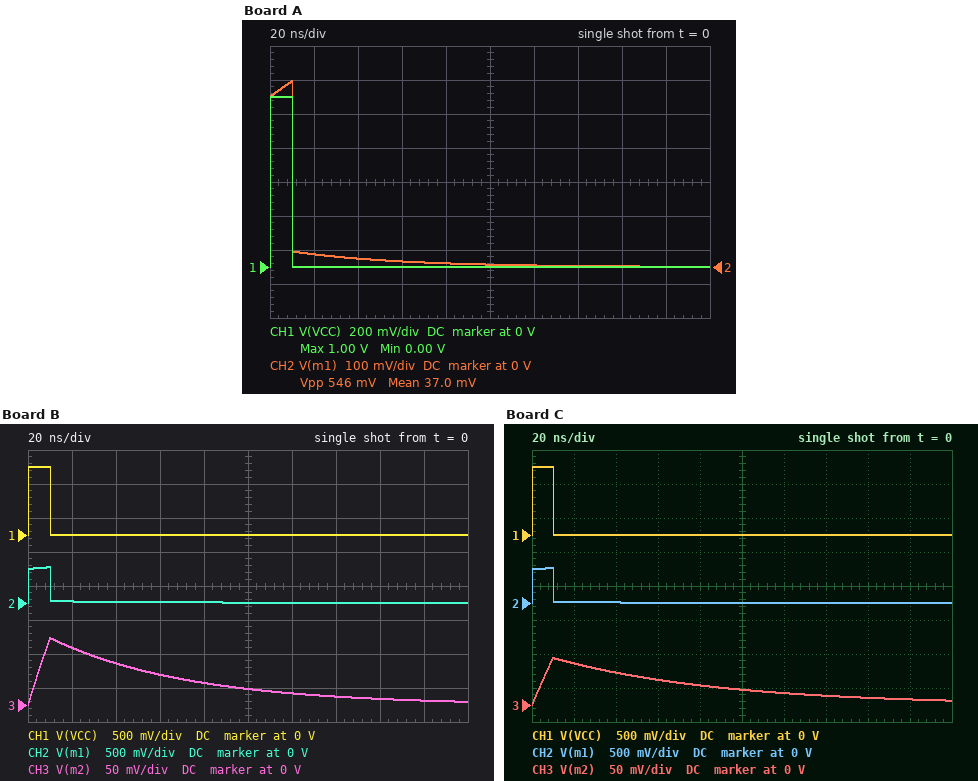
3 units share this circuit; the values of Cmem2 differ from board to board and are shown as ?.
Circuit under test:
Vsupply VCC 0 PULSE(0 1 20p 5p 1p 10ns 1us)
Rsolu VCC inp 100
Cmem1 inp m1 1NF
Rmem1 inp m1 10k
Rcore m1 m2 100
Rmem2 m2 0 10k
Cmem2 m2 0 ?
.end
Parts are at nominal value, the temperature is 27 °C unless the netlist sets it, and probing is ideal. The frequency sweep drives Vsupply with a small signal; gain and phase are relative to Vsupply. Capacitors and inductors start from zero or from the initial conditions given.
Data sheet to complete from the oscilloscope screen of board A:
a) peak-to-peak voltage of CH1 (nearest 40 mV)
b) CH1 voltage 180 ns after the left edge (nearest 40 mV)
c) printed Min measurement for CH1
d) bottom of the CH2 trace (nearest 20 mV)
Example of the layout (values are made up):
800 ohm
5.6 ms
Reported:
1.00 V
0 V
0.00 V
0 V
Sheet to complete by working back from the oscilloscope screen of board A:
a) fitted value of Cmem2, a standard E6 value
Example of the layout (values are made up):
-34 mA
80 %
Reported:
330 pF
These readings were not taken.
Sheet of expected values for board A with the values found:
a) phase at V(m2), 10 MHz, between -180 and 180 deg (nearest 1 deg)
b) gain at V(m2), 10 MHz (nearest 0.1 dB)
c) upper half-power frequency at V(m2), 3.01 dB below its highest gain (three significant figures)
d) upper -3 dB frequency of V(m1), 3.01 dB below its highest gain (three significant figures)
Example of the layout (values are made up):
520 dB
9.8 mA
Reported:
-72 deg
-12.8 dB
3.28 MHz
10.2 MHz
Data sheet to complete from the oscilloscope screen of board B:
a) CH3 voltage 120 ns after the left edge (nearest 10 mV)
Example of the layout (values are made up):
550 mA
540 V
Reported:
20 mV
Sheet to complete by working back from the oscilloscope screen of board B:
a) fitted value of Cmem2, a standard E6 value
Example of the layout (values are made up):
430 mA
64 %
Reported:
470 pF
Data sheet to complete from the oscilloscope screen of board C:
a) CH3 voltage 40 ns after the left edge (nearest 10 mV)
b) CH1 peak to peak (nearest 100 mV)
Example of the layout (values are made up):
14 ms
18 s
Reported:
50 mV
1.0 V
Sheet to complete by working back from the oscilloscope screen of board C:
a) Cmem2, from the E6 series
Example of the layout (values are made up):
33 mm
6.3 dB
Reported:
680 pF
